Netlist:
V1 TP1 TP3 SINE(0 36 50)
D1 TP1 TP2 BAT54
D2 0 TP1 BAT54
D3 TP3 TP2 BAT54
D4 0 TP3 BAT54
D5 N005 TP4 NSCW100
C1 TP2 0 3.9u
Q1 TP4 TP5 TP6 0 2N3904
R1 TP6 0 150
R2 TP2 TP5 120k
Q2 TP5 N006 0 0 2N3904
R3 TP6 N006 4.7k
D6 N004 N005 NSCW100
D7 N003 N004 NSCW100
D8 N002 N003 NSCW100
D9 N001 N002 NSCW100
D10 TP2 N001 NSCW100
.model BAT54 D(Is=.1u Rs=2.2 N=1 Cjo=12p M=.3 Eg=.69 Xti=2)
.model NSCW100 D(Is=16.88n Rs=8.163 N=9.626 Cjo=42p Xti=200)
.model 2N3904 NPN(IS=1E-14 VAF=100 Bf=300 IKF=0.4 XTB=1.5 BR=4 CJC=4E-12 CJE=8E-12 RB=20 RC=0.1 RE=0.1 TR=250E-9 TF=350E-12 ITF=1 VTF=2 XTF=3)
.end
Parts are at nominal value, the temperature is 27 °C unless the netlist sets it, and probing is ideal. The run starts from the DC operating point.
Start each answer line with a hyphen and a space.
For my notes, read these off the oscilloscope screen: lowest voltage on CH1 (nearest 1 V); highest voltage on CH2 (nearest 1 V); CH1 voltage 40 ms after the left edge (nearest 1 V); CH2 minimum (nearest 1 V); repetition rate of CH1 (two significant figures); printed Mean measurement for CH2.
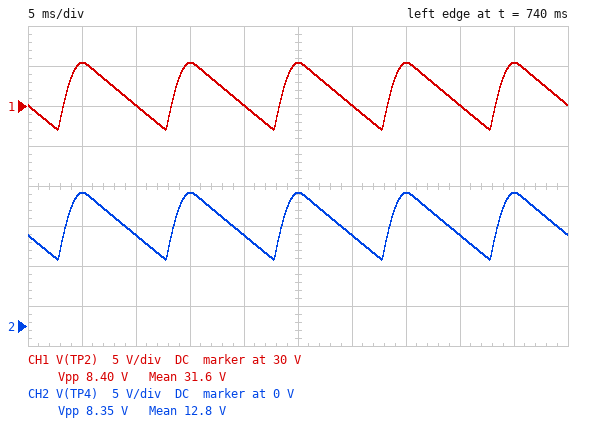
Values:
- 27 V
- 17 V
- 30 V
- 8 V
- 100 Hz
- 12.8 V
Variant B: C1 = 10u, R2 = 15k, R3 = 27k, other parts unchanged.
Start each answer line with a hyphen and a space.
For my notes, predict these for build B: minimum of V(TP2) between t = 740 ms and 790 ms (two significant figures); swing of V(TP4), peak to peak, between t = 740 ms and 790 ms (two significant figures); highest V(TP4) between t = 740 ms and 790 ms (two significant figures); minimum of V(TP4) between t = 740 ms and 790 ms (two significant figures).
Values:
- 29 V
- 6.0 V
- 16 V
- 10 V
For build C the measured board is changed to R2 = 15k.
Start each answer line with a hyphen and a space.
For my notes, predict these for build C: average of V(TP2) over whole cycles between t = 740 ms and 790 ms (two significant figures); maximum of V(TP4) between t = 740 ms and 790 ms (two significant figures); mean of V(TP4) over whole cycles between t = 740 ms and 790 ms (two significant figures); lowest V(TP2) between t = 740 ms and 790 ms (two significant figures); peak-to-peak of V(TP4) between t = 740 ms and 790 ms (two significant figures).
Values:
- 30 V
- 16 V
- 11 V
- 24 V
- 12 V
